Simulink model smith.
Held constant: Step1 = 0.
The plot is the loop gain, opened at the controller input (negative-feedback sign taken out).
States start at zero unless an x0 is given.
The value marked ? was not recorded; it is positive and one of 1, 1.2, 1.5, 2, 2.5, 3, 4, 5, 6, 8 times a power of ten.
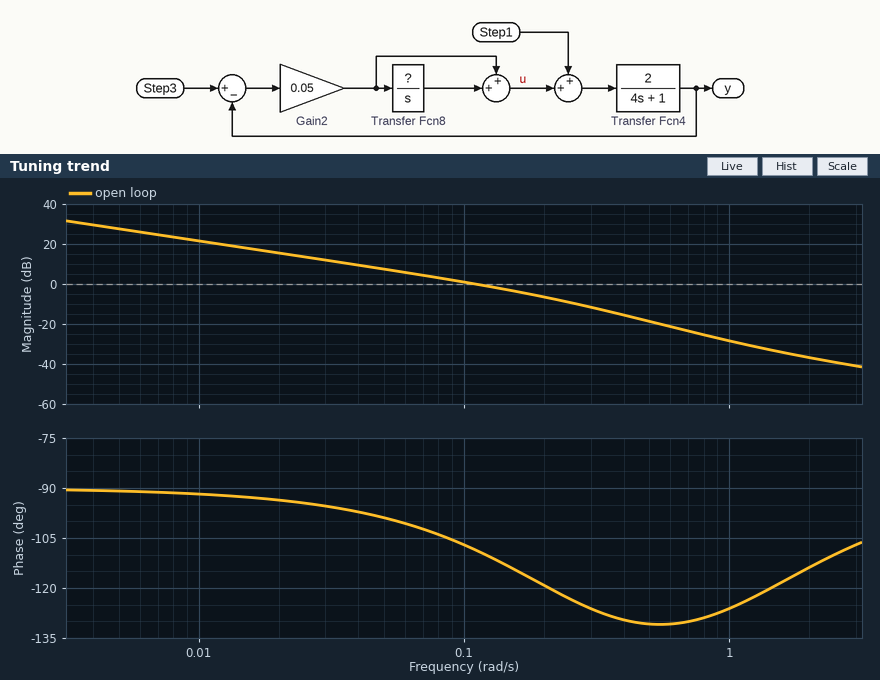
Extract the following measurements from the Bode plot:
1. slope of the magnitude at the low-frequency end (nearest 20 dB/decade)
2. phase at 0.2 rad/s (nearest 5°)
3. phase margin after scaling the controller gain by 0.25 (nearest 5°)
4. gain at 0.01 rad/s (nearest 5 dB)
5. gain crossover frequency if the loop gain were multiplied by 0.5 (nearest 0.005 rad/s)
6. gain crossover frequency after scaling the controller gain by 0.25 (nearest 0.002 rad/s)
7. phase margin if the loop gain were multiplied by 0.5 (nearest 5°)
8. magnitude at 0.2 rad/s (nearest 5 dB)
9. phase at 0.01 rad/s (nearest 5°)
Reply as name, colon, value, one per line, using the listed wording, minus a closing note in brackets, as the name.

slope of the magnitude at the low-frequency end: -20 dB/decade
phase at 0.2 rad/s: -120°
phase margin after scaling the controller gain by 0.25: 85°
gain at 0.01 rad/s: 20 dB
gain crossover frequency if the loop gain were multiplied by 0.5: 0.060 rad/s
gain crossover frequency after scaling the controller gain by 0.25: 0.030 rad/s
phase margin if the loop gain were multiplied by 0.5: 80°
magnitude at 0.2 rad/s: -5 dB
phase at 0.01 rad/s: -90°
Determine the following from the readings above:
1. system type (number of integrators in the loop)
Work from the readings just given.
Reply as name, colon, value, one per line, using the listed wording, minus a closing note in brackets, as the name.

system type: 1
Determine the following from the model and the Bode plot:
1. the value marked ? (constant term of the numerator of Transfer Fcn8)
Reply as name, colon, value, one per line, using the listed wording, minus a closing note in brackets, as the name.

the value marked ?: 1.2
